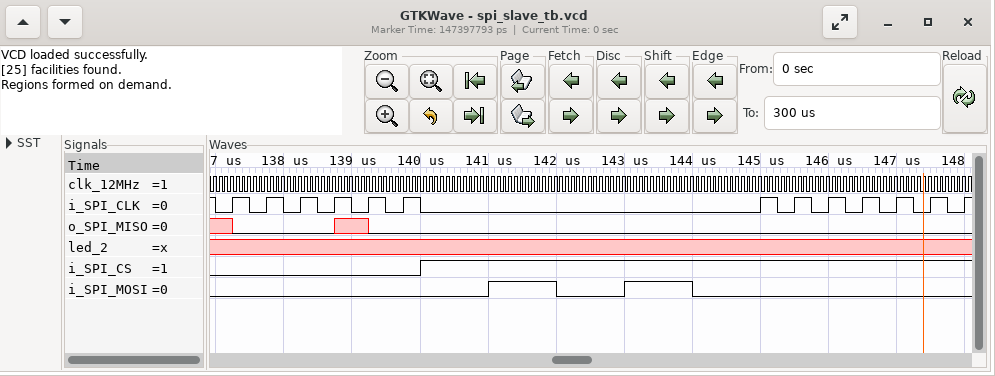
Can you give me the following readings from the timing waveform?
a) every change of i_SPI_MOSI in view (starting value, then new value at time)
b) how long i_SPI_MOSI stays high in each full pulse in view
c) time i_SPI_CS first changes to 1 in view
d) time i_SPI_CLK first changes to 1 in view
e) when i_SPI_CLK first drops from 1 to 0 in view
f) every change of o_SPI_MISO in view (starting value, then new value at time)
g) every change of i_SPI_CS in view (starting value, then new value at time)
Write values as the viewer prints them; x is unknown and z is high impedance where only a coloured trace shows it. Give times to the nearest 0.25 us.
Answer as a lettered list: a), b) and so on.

a) 0, 1 at 141 us, 0 at 142 us, 1 at 143 us, 0 at 144 us
b) 1 us, 1 us
c) 140 us
d) 137.25 us
e) 137 us
f) x, 0 at 137.25 us, x at 138.75 us, 0 at 139.25 us
g) 0, 1 at 140 us
